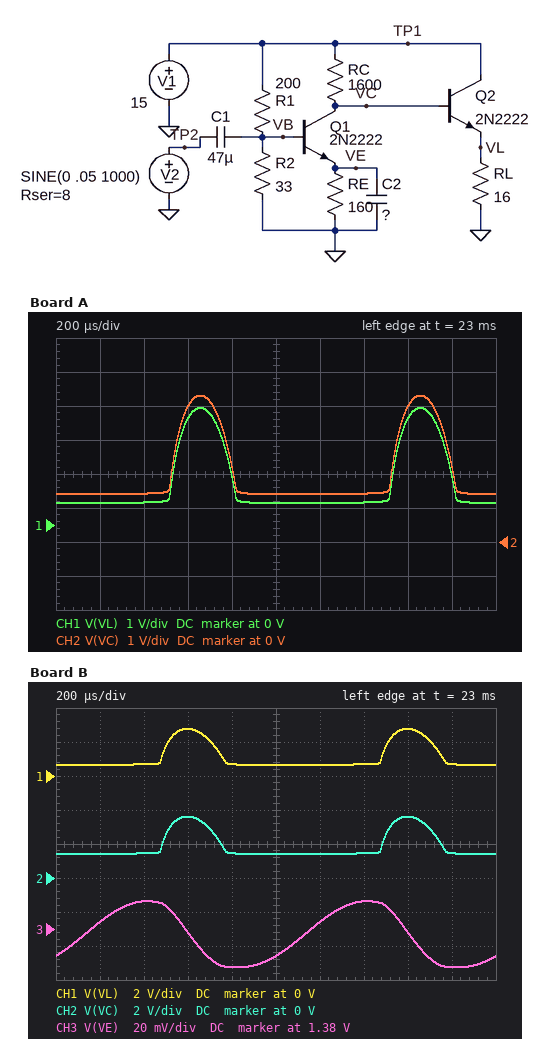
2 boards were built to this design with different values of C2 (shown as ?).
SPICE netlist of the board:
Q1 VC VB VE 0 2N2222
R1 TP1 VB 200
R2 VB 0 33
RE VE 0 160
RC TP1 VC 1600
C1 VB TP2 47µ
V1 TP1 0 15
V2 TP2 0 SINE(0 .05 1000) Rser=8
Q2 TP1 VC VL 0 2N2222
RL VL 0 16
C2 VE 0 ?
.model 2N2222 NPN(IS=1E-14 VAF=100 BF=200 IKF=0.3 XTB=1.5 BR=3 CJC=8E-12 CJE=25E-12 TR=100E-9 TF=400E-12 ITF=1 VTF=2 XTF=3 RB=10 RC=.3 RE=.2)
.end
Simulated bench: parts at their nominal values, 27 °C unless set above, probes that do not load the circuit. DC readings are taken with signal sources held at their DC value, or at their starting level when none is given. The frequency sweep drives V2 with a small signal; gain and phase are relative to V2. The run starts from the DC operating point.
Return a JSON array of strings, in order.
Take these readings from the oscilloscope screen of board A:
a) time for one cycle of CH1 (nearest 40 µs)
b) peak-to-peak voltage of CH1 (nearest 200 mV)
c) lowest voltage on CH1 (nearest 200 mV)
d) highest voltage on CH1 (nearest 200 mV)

["1.00 ms", "2.8 V", "600 mV", "3.4 V"]
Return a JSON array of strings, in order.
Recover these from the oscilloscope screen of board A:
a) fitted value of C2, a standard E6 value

["33 µF"]
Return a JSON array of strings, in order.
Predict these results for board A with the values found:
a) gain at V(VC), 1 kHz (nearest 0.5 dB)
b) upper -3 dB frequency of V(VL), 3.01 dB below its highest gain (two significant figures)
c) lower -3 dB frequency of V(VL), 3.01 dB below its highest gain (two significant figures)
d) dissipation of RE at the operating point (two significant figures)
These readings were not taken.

["3.5 dB", "760 kHz", "320 Hz", "12 mW"]
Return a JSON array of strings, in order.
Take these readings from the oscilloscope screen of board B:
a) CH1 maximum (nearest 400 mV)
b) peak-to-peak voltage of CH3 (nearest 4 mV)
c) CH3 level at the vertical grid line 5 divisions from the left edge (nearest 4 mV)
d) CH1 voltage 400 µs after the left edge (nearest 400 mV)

["2.8 V", "40 mV", "1.364 V", "800 mV"]
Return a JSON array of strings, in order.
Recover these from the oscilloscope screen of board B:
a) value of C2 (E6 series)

["15 µF"]
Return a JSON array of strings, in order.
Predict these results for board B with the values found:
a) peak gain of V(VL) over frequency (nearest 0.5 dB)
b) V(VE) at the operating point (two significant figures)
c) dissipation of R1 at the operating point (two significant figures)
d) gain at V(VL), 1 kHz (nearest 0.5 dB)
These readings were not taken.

["3.5 dB", "1.4 V", "830 mW", "2.5 dB"]
